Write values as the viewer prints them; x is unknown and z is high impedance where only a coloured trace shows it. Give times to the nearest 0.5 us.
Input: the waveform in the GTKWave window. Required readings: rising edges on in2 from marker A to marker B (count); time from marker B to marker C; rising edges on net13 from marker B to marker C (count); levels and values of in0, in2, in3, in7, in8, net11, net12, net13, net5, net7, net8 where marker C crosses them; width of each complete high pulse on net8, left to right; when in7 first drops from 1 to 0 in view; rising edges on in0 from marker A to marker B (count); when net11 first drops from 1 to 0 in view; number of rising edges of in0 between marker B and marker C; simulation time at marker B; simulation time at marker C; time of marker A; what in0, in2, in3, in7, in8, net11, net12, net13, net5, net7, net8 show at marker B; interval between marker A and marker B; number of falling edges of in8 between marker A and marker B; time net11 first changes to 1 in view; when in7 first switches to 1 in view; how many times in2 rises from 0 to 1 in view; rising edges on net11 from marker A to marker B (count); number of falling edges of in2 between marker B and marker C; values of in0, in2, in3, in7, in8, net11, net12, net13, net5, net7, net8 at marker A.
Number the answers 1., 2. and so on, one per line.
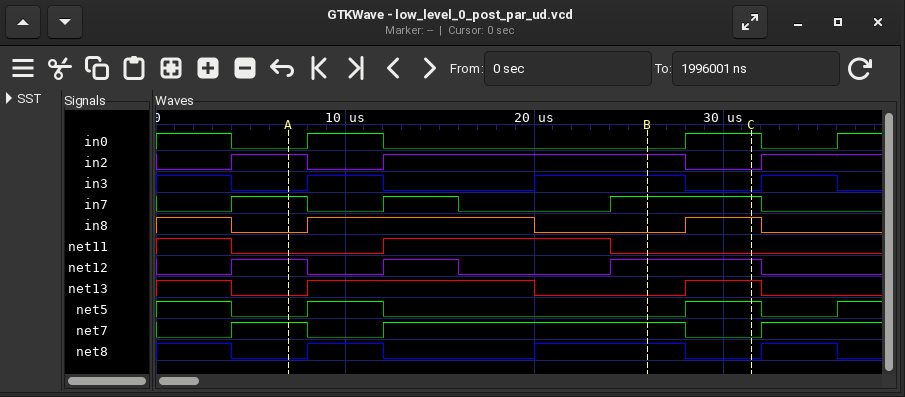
1. 1
2. 5.5 us
3. 1
4. in0=1, in2=0, in3=0, in7=1, in8=1, net11=0, net12=1, net13=1, net5=1, net7=0, net8=0
5. 4 us, 8 us, 4 us
6. 8 us
7. 1
8. 4 us
9. 1
10. 26 us
11. 31.5 us
12. 7 us
13. in0=0, in2=1, in3=1, in7=1, in8=0, net11=0, net12=1, net13=0, net5=0, net7=1, net8=1
14. 19 us
15. 1
16. 12 us
17. 4 us
18. 3
19. 1
20. 1
21. in0=0, in2=1, in3=0, in7=1, in8=0, net11=0, net12=1, net13=0, net5=0, net7=1, net8=0
